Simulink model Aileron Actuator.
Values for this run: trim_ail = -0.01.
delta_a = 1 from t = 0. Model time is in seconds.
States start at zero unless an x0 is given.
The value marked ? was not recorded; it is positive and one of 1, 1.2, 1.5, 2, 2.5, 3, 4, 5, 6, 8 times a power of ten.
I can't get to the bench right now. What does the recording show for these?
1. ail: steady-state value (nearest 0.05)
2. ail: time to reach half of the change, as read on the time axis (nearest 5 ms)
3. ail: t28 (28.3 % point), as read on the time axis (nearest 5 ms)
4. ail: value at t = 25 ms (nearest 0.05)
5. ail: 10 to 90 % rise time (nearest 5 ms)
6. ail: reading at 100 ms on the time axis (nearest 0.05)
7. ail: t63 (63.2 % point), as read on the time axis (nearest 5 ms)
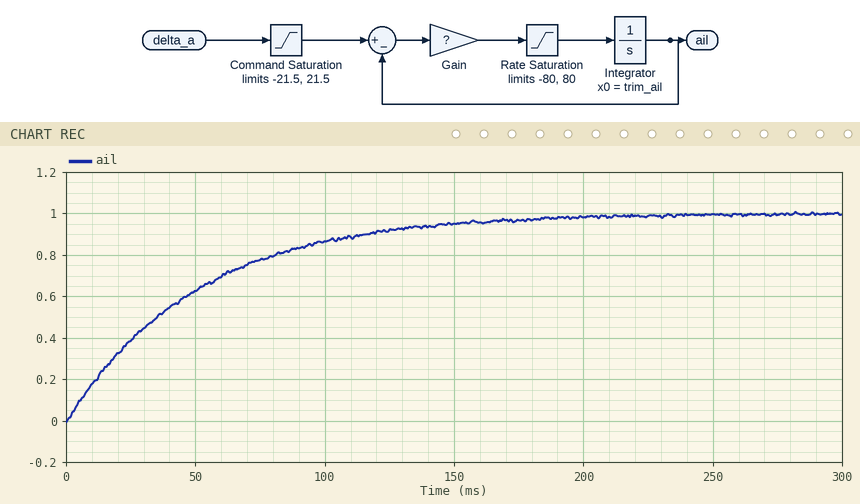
1.00
35 ms
15 ms
0.40
110 ms
0.85
50 ms
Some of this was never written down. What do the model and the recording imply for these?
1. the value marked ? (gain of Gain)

20
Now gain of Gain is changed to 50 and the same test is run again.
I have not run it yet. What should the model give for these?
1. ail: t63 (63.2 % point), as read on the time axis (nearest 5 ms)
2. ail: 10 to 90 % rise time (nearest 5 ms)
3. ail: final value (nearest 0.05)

20 ms
45 ms
1.00
